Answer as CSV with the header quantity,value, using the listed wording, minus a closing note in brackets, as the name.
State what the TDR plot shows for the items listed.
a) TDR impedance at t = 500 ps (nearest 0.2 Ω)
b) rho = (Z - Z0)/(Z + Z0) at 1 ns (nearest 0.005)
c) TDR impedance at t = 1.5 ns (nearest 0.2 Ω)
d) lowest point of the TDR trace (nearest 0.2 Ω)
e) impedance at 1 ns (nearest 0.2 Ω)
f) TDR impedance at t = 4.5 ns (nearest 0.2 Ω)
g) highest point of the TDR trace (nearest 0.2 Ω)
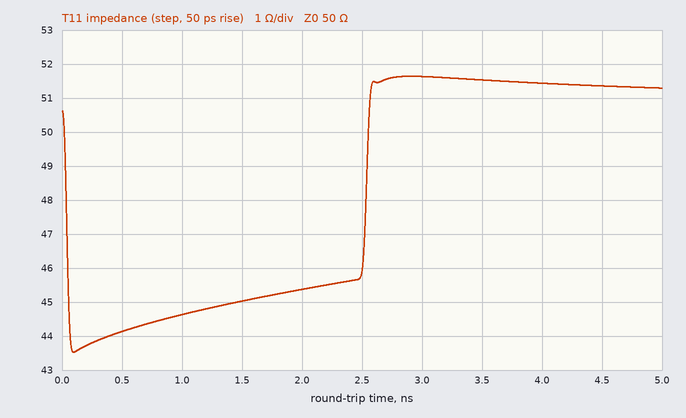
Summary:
quantity,value
TDR impedance at t = 500 ps,44.2 Ω
rho = (Z - Z0)/(Z + Z0) at 1 ns,-0.055
TDR impedance at t = 1.5 ns,45.0 Ω
lowest point of the TDR trace,43.6 Ω
impedance at 1 ns,44.6 Ω
TDR impedance at t = 4.5 ns,51.4 Ω
highest point of the TDR trace,51.6 Ω
